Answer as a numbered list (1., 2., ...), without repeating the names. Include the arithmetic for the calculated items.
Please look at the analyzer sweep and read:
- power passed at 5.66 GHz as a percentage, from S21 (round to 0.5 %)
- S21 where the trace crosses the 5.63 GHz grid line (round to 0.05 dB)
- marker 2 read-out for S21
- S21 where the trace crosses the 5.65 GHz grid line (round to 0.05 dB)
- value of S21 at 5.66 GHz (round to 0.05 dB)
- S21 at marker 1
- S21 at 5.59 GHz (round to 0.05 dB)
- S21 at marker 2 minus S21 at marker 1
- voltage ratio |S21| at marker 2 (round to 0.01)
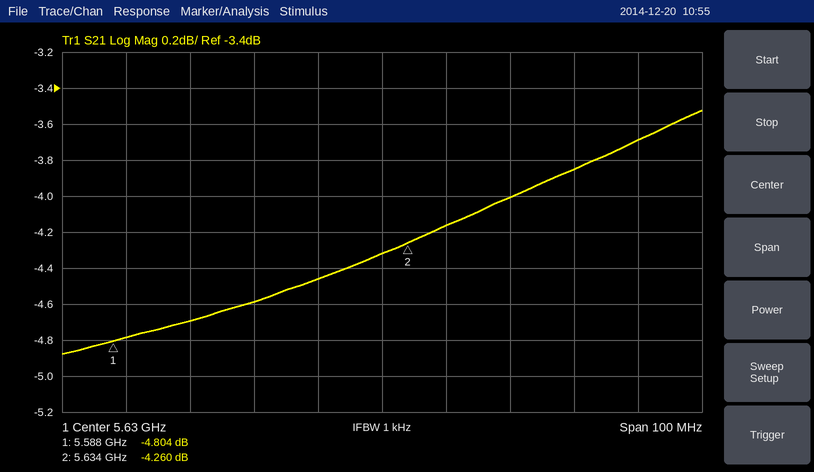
1. 10^(-3.85/10) ≈ 41.2 %, so 41.0 % to the nearest 0.5 %
2. -4.30 dB
3. -4.260 dB
4. -4.00 dB
5. -3.85 dB
6. -4.804 dB
7. -4.80 dB
8. -4.26 − (-4.804) = 0.544 dB
9. 10^(-4.26/20) ≈ 0.61
